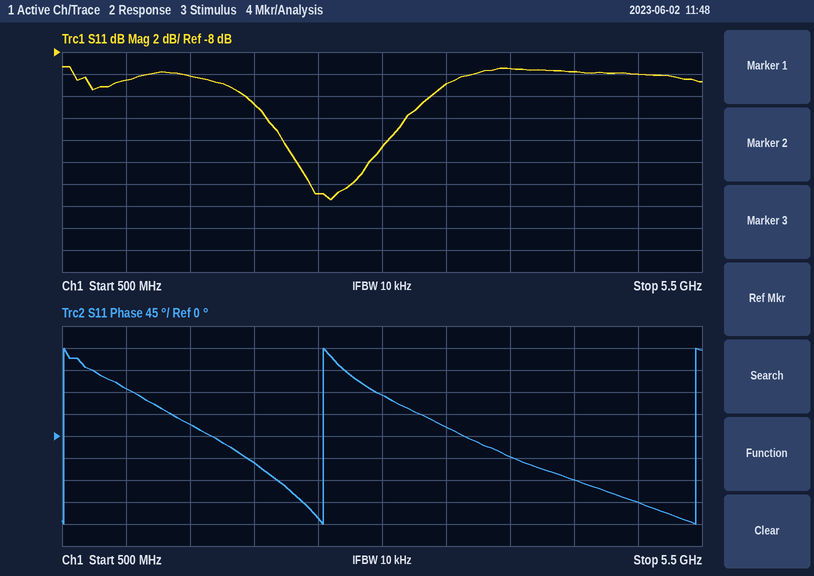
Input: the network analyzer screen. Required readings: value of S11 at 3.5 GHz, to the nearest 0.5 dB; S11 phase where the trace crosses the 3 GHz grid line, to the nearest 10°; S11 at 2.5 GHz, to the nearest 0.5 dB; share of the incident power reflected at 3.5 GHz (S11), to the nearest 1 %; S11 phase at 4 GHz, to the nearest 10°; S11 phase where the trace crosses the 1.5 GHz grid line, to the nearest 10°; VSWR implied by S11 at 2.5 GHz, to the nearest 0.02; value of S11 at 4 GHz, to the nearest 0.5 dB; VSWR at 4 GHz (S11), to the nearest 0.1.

-11.0 dB
80°
-21.0 dB
8 %
-40°
20°
1.20
-9.5 dB
2.0
